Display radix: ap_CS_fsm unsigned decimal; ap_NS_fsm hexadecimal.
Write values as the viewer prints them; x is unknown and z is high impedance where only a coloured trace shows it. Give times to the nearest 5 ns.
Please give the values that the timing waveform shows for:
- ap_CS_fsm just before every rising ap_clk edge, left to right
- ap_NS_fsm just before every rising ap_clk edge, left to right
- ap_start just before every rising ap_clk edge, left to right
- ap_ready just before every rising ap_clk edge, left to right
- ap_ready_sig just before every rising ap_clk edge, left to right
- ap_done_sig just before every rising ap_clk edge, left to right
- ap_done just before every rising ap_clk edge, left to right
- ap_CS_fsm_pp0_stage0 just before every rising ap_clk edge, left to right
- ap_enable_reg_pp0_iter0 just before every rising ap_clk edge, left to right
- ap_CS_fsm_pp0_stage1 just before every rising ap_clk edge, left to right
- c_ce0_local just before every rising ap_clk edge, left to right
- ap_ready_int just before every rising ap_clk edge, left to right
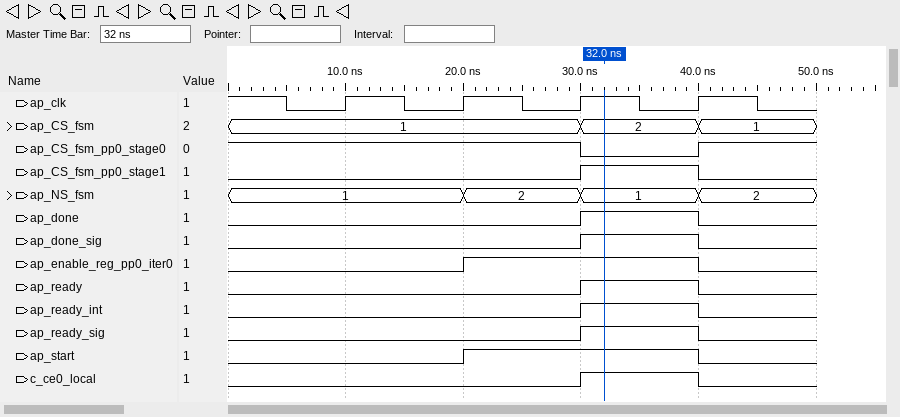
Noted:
1, 1, 1, 2
1, 1, 2, 1
0 0 1 1
0 0 0 1
0 0 0 1
0 0 0 1
0 0 0 1
1 1 1 0
0 0 1 1
0 0 0 1
0 0 0 1
0 0 0 1
